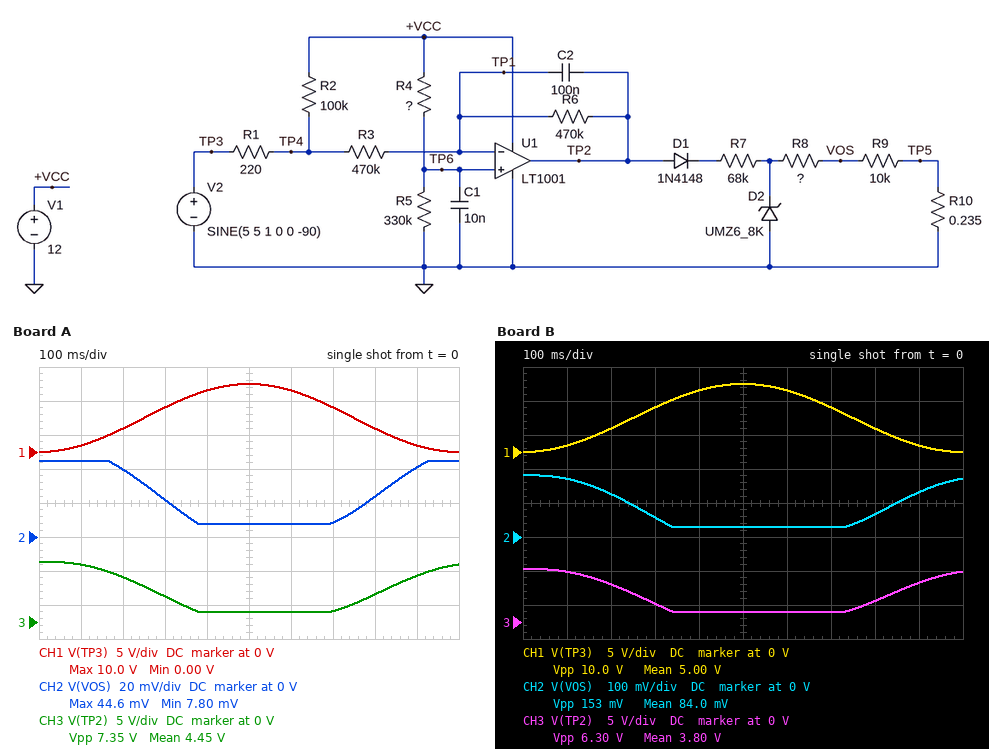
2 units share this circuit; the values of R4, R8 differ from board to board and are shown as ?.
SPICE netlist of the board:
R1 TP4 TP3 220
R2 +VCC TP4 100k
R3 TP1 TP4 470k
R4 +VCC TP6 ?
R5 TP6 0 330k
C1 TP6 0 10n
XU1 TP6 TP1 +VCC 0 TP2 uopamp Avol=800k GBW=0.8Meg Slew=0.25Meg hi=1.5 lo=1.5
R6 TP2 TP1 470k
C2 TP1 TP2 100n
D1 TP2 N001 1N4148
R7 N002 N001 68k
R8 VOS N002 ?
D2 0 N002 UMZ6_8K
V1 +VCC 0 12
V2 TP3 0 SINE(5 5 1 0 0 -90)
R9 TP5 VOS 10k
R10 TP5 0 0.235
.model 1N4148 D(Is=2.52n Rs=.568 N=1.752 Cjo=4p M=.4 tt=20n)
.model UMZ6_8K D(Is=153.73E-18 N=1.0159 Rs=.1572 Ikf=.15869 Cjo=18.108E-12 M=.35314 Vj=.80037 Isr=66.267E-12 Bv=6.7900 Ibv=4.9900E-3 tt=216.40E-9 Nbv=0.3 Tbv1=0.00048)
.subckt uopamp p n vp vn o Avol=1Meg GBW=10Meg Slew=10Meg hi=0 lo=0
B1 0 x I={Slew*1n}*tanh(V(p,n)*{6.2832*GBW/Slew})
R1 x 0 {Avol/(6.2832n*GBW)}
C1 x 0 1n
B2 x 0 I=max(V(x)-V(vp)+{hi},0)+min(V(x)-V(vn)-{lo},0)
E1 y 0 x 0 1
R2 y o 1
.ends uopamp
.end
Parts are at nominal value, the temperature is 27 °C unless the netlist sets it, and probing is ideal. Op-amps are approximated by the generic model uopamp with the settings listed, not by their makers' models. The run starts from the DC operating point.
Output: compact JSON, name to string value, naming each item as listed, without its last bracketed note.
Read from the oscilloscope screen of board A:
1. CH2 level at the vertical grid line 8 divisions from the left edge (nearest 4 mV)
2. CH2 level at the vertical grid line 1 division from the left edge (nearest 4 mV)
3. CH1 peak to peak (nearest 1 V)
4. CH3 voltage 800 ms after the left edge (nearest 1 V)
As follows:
{"CH2 level at the vertical grid line 8 divisions from the left edge": "24 mV", "CH2 level at the vertical grid line 1 division from the left edge": "44 mV", "CH1 peak to peak": "10 V", "CH3 voltage 800 ms after the left edge": "4 V"}
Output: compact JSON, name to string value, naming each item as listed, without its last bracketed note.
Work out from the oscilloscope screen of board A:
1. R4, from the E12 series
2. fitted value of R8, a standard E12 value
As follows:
{"R4, from the E12 series": "560 kΩ", "fitted value of R8, a standard E12 value": "1.5 MΩ"}
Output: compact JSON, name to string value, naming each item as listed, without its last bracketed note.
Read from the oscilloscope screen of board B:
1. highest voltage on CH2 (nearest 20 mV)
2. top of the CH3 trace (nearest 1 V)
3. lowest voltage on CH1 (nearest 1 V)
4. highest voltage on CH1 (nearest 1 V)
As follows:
{"highest voltage on CH2": "180 mV", "top of the CH3 trace": "8 V", "lowest voltage on CH1": "0 V", "highest voltage on CH1": "10 V"}
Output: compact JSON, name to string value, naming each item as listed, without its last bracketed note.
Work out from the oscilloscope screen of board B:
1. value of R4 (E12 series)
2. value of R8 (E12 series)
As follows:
{"value of R4": "680 kΩ", "value of R8": "330 kΩ"}
